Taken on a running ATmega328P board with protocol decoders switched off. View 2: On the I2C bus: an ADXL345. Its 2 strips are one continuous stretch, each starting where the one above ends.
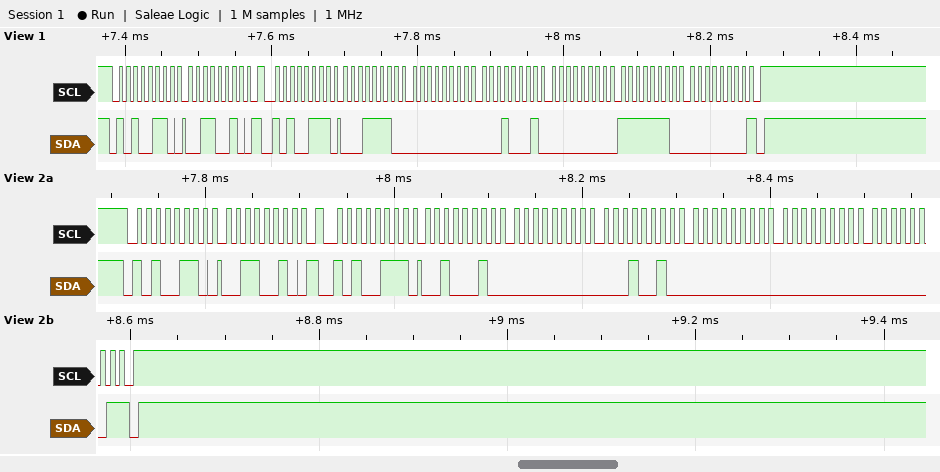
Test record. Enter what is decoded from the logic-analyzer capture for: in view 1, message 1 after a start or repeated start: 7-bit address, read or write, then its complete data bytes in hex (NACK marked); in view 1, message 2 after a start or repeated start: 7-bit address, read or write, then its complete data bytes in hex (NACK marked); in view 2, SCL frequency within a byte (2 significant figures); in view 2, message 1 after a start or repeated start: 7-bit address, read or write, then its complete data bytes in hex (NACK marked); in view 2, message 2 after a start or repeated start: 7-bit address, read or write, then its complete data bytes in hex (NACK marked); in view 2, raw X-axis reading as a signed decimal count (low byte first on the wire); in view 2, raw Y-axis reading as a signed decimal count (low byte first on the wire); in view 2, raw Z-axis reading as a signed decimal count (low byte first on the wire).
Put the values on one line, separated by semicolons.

0x53 write: 32; 0x53 read: 1E 00 11 00 FE 00 NACK; 100 kHz; 0x53 write: 32; 0x53 read: 22 00 12 00 00 01 NACK; 34; 18; 256
